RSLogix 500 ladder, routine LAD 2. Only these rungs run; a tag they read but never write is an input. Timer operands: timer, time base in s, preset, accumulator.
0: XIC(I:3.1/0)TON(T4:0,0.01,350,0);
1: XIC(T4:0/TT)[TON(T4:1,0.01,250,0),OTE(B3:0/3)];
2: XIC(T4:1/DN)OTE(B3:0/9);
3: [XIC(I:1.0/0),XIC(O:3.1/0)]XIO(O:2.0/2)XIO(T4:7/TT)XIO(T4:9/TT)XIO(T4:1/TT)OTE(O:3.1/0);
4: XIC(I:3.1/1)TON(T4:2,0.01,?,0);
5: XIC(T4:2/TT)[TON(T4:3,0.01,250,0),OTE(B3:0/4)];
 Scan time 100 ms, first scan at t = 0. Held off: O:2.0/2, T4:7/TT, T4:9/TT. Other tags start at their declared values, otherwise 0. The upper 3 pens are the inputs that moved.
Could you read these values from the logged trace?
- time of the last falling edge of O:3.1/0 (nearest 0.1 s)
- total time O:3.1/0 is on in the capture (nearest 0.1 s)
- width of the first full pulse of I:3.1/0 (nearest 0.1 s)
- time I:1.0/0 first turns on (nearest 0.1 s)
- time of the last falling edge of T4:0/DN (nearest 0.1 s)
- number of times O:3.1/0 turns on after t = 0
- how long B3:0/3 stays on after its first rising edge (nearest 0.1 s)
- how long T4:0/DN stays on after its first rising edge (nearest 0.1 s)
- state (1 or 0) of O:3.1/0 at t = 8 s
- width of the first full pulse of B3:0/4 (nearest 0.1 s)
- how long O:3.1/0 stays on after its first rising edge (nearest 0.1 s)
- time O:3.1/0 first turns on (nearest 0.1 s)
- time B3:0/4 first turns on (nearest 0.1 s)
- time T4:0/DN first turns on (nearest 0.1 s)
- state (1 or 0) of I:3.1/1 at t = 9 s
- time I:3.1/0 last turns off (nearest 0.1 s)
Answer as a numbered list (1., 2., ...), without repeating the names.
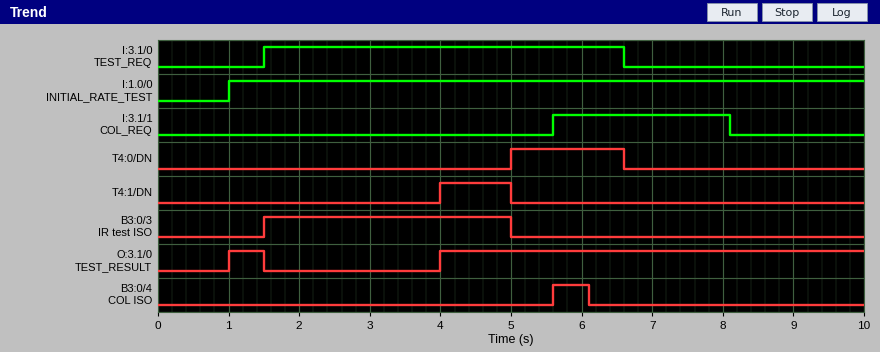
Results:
1. 1.5 s
2. 6.5 s
3. 5.1 s
4. 1.0 s
5. 6.6 s
6. 2
7. 3.5 s
8. 1.6 s
9. 1
10. 0.5 s
11. 0.5 s
12. 1.0 s
13. 5.6 s
14. 5.0 s
15. 0
16. 6.6 s
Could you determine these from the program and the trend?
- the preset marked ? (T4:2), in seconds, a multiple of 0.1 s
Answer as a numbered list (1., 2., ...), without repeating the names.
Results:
1. 0.5 s
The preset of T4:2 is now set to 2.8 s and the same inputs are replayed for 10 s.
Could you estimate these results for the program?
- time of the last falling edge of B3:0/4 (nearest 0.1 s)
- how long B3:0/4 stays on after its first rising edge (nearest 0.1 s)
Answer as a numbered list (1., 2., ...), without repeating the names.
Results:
1. 8.1 s
2. 2.5 s
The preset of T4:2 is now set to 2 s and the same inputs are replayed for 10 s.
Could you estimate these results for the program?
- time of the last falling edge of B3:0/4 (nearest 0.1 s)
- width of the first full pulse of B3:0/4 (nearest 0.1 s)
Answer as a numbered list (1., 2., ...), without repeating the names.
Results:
1. 7.6 s
2. 2.0 s
